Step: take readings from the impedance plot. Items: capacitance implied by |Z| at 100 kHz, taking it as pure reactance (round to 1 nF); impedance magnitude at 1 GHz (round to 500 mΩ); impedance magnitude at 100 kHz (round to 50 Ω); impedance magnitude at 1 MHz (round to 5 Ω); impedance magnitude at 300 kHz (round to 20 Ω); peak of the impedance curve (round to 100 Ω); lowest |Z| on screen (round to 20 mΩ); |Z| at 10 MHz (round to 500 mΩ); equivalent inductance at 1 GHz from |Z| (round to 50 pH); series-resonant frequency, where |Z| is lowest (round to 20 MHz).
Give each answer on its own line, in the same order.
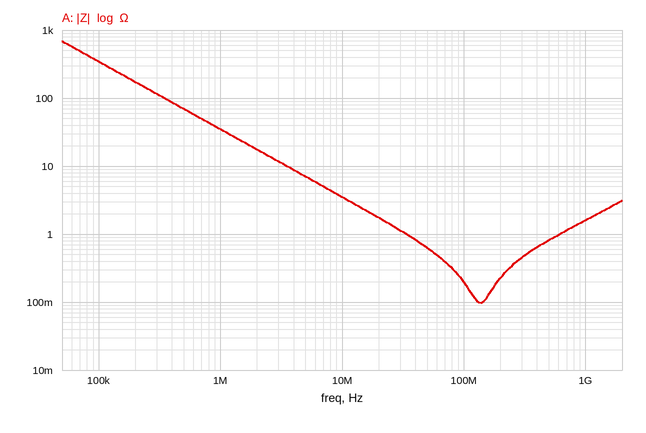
5 nF
1.5 Ω
350 Ω
35 Ω
120 Ω
700 Ω
100 mΩ
3.5 Ω
250 pH
140 MHz
